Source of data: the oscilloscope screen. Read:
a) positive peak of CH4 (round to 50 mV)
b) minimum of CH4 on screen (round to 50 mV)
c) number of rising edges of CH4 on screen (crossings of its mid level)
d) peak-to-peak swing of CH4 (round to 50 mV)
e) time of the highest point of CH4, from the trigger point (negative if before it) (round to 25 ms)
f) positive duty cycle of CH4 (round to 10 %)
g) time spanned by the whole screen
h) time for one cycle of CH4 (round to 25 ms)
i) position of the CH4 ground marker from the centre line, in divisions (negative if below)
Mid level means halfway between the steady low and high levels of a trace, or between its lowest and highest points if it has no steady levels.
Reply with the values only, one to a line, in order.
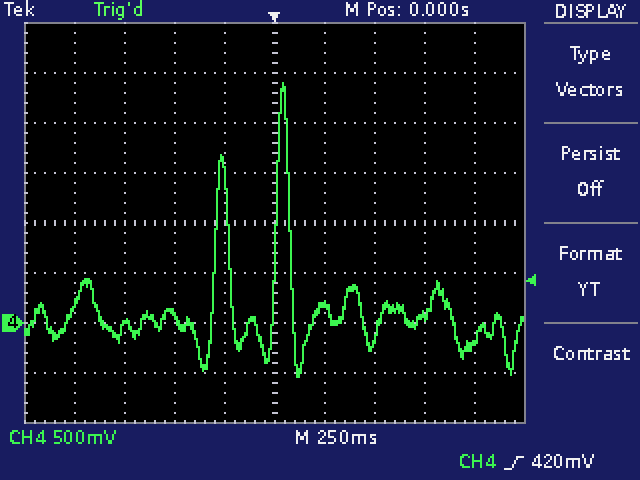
2.40 V
-550 mV
2
2.95 V
+50 ms
20 %
2.5 s
300 ms
-2.0 div
